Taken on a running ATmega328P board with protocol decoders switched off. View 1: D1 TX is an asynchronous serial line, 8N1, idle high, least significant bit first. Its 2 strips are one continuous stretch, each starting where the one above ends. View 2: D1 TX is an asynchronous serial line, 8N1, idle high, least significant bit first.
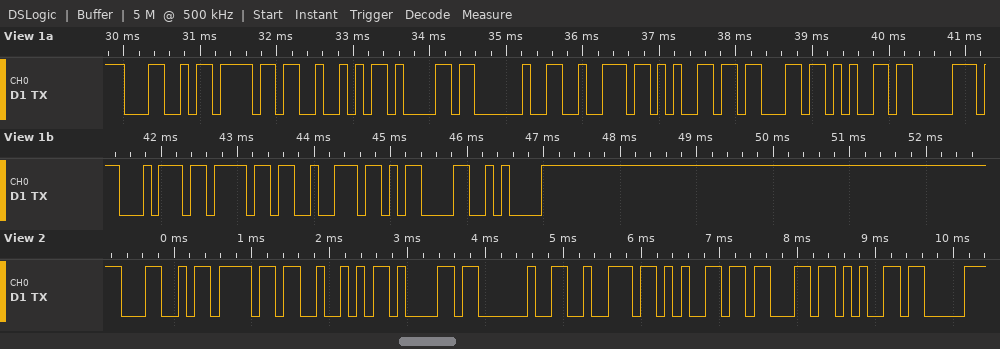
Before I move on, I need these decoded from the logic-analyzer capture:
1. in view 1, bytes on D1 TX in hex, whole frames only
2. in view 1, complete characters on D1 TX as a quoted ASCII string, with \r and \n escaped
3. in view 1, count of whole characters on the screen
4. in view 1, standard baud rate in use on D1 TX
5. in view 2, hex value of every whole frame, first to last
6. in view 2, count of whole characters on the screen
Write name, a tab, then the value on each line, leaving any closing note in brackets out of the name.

in view 1, bytes on D1 TX in hex, whole frames only	4C 6F 52 61 20 72 65 63 65 70 74 6F 72 0D 0A
in view 1, complete characters on D1 TX as a quoted ASCII string, with \r and \n escaped	"LoRa receptor\r\n"
in view 1, count of whole characters on the screen	15
in view 1, standard baud rate in use on D1 TX	9600 baud
in view 2, hex value of every whole frame, first to last	0x4C 0x6F 0x52 0x61 0x20 0x72 0x65 0x63 0x65
in view 2, count of whole characters on the screen	9
